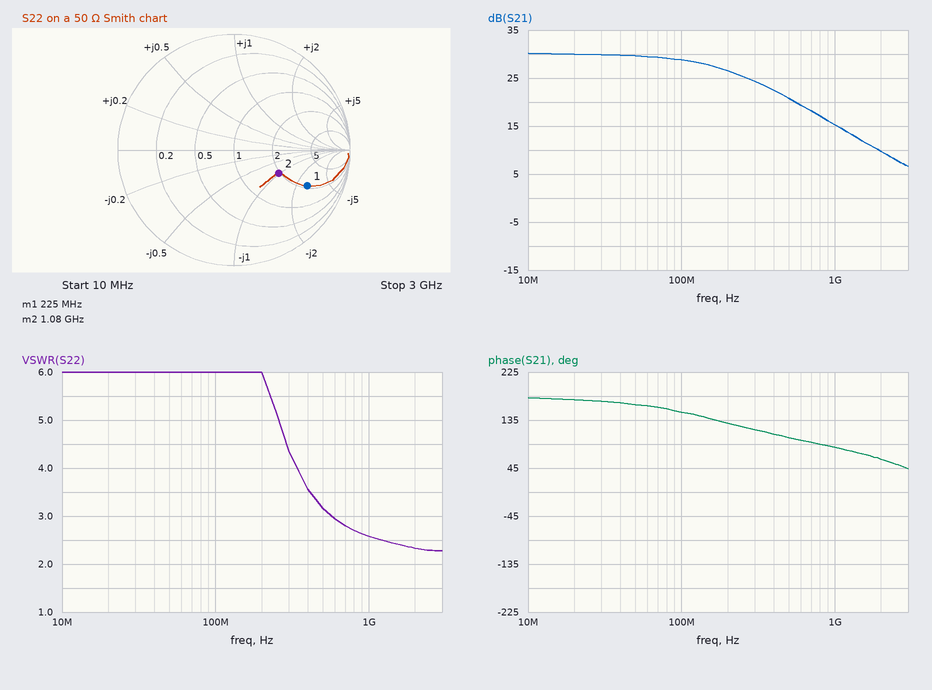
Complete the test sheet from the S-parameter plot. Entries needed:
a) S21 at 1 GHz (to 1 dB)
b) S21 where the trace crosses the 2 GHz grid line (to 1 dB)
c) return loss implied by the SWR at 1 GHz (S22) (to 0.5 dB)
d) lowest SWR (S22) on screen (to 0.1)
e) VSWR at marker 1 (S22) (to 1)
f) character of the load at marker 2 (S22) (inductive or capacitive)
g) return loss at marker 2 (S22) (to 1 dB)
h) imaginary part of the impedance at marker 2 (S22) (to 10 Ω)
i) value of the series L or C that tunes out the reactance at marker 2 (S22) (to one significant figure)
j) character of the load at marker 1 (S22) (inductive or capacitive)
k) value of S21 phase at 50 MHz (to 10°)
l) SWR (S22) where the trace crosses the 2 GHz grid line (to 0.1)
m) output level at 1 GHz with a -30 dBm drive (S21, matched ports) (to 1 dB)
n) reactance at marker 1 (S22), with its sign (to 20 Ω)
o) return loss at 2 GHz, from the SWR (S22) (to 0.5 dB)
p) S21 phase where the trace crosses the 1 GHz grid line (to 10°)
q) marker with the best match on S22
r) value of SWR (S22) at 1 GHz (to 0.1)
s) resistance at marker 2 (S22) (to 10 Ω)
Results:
15 dB
10 dB
7.0 dB
2.3
6
capacitive
7 dB
-50 Ω
7 nH
capacitive
160°
2.3
-15 dBm
-140 Ω
8.0 dB
80°
marker 2
2.6
100 Ω
